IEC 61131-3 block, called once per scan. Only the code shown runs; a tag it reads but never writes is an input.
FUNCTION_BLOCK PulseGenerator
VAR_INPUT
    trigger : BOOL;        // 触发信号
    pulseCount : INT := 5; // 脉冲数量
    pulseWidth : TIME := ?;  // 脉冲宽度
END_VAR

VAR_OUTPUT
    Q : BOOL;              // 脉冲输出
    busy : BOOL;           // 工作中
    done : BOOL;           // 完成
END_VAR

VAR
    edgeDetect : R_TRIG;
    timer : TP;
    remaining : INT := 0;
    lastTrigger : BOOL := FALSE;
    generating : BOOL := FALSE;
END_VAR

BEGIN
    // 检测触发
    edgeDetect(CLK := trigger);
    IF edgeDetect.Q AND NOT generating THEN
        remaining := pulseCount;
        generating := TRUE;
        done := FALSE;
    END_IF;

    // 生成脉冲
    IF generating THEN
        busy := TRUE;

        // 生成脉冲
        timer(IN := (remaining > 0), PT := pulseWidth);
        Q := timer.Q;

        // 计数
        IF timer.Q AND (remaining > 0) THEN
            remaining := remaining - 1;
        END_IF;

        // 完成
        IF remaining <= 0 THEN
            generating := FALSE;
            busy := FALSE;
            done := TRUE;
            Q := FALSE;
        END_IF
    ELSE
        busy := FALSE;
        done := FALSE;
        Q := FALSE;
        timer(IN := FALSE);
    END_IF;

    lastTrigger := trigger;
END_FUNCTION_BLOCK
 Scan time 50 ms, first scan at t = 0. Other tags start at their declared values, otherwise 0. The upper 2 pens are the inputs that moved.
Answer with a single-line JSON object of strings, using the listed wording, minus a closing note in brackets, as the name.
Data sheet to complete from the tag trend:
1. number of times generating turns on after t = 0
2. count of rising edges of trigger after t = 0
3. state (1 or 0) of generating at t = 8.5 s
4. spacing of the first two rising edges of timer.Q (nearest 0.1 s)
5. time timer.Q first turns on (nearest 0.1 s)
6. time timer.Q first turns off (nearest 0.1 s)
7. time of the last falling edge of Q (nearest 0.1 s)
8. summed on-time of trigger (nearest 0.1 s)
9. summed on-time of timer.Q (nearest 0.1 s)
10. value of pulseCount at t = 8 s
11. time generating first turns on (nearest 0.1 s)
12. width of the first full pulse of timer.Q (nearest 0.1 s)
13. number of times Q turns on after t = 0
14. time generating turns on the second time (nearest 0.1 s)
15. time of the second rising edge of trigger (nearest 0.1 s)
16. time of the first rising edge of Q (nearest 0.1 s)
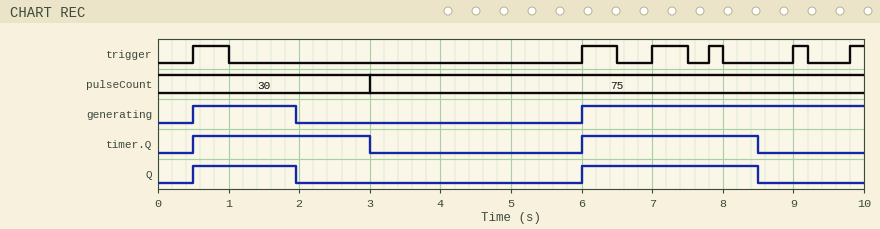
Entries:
{"number of times generating turns on after t = 0": "2", "count of rising edges of trigger after t = 0": "6", "state (1 or 0) of generating at t = 8.5 s": "1", "spacing of the first two rising edges of timer.Q": "5.5 s", "time timer.Q first turns on": "0.5 s", "time timer.Q first turns off": "3.0 s", "time of the last falling edge of Q": "8.5 s", "summed on-time of trigger": "2.1 s", "summed on-time of timer.Q": "5.0 s", "value of pulseCount at t = 8 s": "75", "time generating first turns on": "0.5 s", "width of the first full pulse of timer.Q": "2.5 s", "number of times Q turns on after t = 0": "2", "time generating turns on the second time": "6.0 s", "time of the second rising edge of trigger": "6.0 s", "time of the first rising edge of Q": "0.5 s"}
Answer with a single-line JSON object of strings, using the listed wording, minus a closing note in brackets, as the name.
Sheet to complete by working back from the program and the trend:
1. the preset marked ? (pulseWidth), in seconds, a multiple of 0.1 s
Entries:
{"the preset marked ? (pulseWidth), in seconds, a multiple of 0.1 s": "2.5 s"}
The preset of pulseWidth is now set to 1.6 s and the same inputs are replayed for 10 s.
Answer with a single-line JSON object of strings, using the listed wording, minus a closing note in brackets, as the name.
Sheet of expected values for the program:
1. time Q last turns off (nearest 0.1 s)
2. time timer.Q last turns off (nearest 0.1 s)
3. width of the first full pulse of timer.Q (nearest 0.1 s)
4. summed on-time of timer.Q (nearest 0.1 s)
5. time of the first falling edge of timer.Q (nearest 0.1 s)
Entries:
{"time Q last turns off": "7.6 s", "time timer.Q last turns off": "7.6 s", "width of the first full pulse of timer.Q": "1.6 s", "summed on-time of timer.Q": "3.2 s", "time of the first falling edge of timer.Q": "2.1 s"}
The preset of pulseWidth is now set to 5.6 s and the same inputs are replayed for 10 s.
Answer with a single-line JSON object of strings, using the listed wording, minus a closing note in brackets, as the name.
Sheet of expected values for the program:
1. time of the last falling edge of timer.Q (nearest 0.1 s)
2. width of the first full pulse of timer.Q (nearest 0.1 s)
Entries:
{"time of the last falling edge of timer.Q": "6.1 s", "width of the first full pulse of timer.Q": "5.6 s"}
